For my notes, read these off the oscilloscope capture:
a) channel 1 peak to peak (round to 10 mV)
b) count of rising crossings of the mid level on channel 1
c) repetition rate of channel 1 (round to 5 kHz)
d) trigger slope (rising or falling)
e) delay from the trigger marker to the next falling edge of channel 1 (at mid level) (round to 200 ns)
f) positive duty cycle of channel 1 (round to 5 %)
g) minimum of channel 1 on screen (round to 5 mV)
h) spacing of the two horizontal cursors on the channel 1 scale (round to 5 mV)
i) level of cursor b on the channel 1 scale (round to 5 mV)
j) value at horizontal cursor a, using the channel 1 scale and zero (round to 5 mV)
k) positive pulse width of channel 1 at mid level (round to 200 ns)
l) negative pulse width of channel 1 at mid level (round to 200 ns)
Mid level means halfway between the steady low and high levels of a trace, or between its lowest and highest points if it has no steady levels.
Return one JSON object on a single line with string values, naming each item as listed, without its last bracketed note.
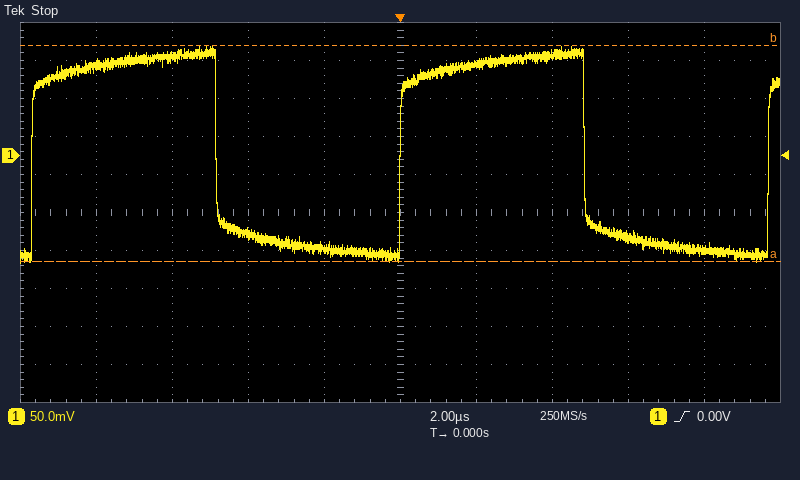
{"channel 1 peak to peak": "280 mV", "count of rising crossings of the mid level on channel 1": "3", "repetition rate of channel 1": "105 kHz", "trigger slope": "rising", "delay from the trigger marker to the next falling edge of channel 1 (at mid level)": "4.8 µs", "positive duty cycle of channel 1": "50 %", "minimum of channel 1 on screen": "-140 mV", "spacing of the two horizontal cursors on the channel 1 scale": "285 mV", "level of cursor b on the channel 1 scale": "145 mV", "value at horizontal cursor a, using the channel 1 scale and zero": "-140 mV", "positive pulse width of channel 1 at mid level": "4.8 µs", "negative pulse width of channel 1 at mid level": "4.8 µs"}
